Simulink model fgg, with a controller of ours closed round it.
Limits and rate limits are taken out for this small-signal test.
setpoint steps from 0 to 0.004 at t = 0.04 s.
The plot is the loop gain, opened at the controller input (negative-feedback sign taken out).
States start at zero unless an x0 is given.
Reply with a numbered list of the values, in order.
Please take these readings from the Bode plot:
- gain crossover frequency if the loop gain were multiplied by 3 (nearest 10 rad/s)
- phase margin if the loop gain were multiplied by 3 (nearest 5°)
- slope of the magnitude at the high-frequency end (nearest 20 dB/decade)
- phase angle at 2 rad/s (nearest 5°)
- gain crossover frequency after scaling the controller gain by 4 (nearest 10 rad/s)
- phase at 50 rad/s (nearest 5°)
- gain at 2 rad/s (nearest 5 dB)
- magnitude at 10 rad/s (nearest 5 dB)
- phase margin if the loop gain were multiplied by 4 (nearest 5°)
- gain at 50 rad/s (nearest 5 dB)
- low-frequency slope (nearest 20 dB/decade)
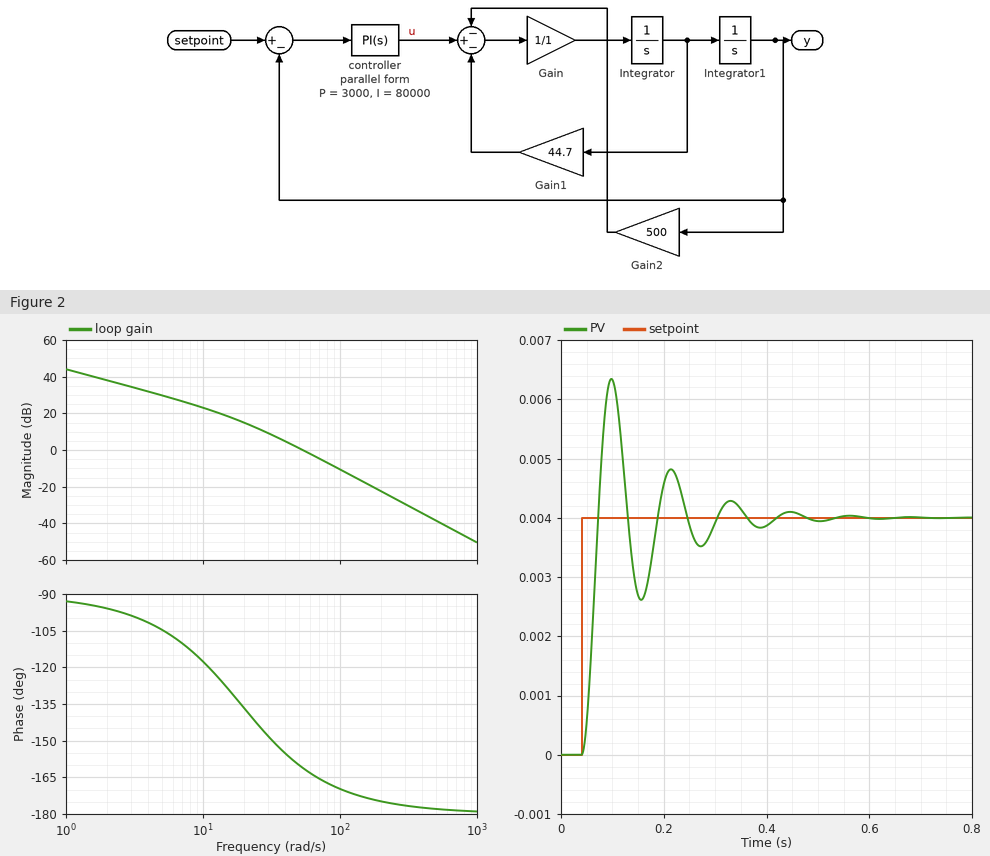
1. 90 rad/s
2. 10°
3. -40 dB/decade
4. -95°
5. 110 rad/s
6. -160°
7. 40 dB
8. 25 dB
9. 10°
10. 0 dB
11. -20 dB/decade
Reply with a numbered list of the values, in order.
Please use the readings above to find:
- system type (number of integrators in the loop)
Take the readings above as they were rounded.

1. 1
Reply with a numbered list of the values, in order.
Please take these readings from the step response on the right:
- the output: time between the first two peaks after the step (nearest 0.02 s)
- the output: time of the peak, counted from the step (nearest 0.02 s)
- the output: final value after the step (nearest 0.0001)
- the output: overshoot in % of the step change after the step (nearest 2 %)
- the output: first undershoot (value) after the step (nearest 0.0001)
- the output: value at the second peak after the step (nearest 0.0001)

1. 0.12 s
2. 0.06 s
3. 0.0040
4. 58 %
5. 0.0026
6. 0.0048
